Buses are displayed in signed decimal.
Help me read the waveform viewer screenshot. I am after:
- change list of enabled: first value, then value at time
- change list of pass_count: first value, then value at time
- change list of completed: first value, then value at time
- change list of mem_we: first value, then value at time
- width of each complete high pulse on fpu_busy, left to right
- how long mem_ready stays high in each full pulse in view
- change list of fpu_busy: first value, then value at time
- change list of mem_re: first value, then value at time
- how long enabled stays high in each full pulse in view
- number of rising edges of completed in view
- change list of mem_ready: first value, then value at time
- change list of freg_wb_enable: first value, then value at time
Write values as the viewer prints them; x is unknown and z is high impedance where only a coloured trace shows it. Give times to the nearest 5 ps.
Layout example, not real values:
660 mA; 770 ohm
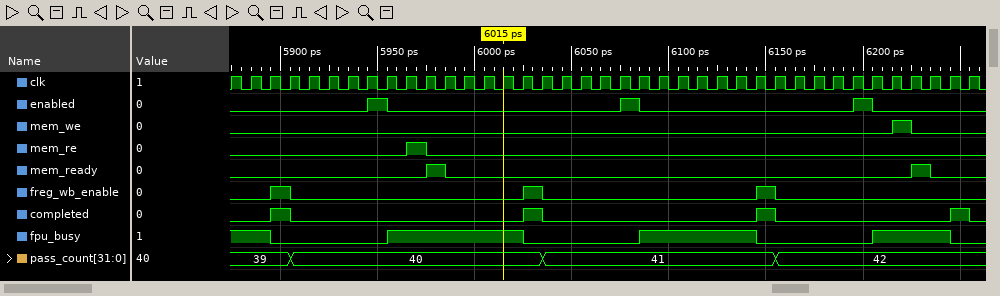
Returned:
0, 1 at 5945 ps, 0 at 5955 ps, 1 at 6075 ps, 0 at 6085 ps, 1 at 6195 ps, 0 at 6205 ps; 39, 40 at 5905 ps, 41 at 6035 ps, 42 at 6155 ps; 0, 1 at 5895 ps, 0 at 5905 ps, 1 at 6025 ps, 0 at 6035 ps, 1 at 6145 ps, 0 at 6155 ps, 1 at 6245 ps, 0 at 6255 ps; 0, 1 at 6215 ps, 0 at 6225 ps; 70 ps, 60 ps, 40 ps; 10 ps, 10 ps; 1, 0 at 5895 ps, 1 at 5955 ps, 0 at 6025 ps, 1 at 6085 ps, 0 at 6145 ps, 1 at 6205 ps, 0 at 6245 ps; 0, 1 at 5965 ps, 0 at 5975 ps; 10 ps, 10 ps, 10 ps; 4; 0, 1 at 5975 ps, 0 at 5985 ps, 1 at 6225 ps, 0 at 6235 ps; 0, 1 at 5895 ps, 0 at 5905 ps, 1 at 6025 ps, 0 at 6035 ps, 1 at 6145 ps, 0 at 6155 ps
